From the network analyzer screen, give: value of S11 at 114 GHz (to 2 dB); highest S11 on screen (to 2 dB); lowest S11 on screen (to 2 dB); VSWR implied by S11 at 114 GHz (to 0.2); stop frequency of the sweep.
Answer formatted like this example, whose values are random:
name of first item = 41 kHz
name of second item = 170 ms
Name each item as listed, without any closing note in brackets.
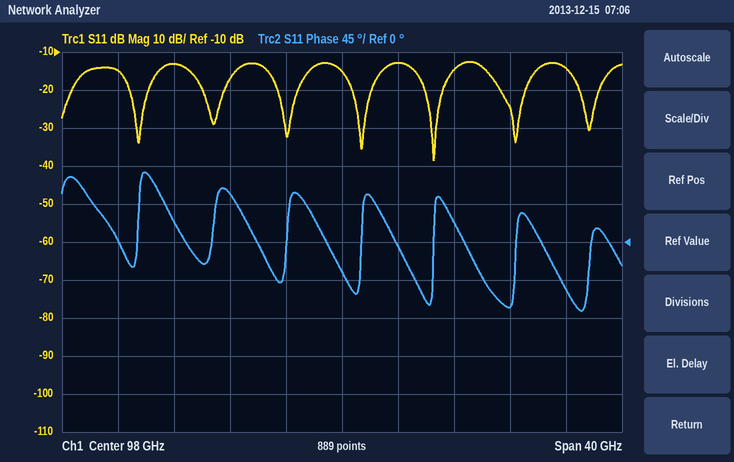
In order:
value of S11 at 114 GHz = -14 dB
highest S11 on screen = -12 dB
lowest S11 on screen = -38 dB
VSWR implied by S11 at 114 GHz = 1.4
stop frequency of the sweep = 118 GHz
